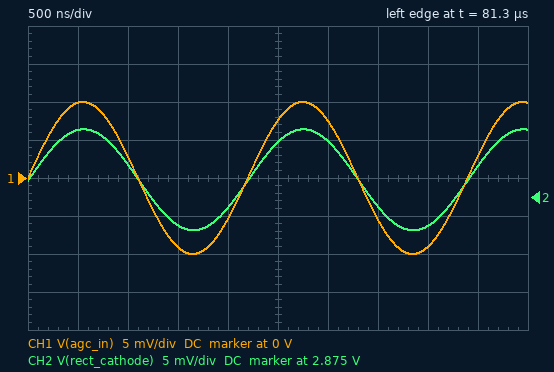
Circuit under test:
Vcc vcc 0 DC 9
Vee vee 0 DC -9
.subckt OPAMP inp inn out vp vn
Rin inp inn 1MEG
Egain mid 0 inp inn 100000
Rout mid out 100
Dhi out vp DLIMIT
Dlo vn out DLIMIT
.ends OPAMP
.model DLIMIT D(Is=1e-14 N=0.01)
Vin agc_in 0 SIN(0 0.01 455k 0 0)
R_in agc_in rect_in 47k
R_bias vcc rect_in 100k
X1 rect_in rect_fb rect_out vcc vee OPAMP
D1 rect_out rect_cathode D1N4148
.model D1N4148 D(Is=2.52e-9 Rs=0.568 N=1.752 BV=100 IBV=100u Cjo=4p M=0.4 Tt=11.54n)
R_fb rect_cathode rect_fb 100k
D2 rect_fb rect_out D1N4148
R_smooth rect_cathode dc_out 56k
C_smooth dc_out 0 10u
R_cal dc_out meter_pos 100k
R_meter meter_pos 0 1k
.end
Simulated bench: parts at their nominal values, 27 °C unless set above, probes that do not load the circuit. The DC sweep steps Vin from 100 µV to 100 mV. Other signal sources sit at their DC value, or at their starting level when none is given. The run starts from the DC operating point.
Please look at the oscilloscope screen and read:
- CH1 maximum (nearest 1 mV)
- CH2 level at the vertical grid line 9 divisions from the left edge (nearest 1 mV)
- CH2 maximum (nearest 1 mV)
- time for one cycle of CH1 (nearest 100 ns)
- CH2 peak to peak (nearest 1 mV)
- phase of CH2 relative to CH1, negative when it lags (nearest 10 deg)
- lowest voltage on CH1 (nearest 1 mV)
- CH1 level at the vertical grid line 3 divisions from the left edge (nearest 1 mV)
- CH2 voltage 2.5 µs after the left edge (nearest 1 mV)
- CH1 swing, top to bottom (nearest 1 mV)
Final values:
10 mV
2.879 V
2.884 V
2.2 µs
13 mV
0 deg
-10 mV
-9 mV
2.882 V
20 mV
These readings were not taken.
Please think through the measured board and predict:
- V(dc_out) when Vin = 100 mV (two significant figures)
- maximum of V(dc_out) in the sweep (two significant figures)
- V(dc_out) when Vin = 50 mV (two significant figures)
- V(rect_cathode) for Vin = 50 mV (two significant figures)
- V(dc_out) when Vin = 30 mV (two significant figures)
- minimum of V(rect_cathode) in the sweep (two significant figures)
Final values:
1.9 V
1.9 V
1.9 V
2.9 V
1.9 V
2.9 V
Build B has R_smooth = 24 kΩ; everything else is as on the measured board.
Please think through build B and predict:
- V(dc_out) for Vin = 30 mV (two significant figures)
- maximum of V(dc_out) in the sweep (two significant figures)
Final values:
2.3 V
2.4 V
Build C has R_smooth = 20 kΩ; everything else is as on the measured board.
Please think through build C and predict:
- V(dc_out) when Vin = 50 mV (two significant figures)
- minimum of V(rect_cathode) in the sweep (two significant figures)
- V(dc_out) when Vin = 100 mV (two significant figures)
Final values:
2.4 V
2.9 V
2.5 V
